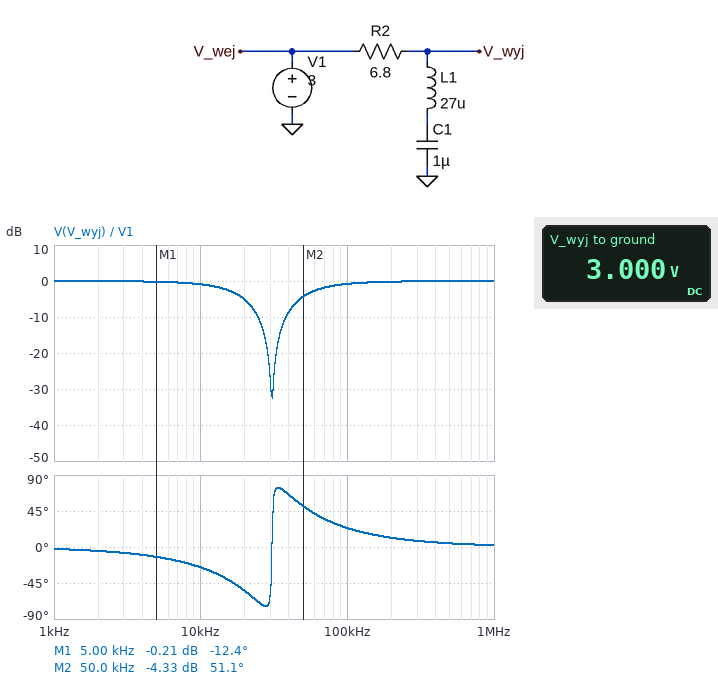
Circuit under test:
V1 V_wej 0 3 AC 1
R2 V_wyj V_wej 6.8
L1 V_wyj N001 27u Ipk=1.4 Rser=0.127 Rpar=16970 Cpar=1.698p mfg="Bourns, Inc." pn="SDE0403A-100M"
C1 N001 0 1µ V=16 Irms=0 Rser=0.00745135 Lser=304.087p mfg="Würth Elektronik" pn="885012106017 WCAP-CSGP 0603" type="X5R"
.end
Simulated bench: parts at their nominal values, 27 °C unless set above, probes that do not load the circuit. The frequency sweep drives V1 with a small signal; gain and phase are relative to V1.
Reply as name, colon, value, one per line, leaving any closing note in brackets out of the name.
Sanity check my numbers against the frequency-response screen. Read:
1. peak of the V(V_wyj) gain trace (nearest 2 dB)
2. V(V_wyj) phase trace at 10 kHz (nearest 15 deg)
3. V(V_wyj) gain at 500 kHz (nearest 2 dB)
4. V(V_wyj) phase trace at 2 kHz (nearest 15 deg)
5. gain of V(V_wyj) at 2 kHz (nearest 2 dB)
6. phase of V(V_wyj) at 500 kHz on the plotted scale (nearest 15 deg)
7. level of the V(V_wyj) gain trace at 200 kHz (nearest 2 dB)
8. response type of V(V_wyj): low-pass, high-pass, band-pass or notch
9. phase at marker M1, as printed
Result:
peak of the V(V_wyj) gain trace: 0 dB
V(V_wyj) phase trace at 10 kHz: -30 deg
V(V_wyj) gain at 500 kHz: 0 dB
V(V_wyj) phase trace at 2 kHz: 0 deg
gain of V(V_wyj) at 2 kHz: 0 dB
phase of V(V_wyj) at 500 kHz on the plotted scale: 0 deg
level of the V(V_wyj) gain trace at 200 kHz: 0 dB
response type of V(V_wyj): low-pass, high-pass, band-pass or notch: notch
phase at marker M1, as printed: -12.4 deg
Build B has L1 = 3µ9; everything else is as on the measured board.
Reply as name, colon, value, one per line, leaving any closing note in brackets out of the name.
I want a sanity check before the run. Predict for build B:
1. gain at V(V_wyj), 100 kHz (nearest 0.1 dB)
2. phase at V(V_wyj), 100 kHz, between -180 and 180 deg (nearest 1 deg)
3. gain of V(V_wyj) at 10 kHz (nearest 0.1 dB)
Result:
gain at V(V_wyj), 100 kHz: -18.1 dB
phase at V(V_wyj), 100 kHz, between -180 and 180 deg: 74 deg
gain of V(V_wyj) at 10 kHz: -0.8 dB
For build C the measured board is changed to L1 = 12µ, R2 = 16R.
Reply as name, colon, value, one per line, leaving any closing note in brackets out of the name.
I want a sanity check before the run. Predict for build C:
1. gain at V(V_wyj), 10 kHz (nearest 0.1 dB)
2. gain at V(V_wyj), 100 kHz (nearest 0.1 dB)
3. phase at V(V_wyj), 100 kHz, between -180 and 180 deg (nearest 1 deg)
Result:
gain at V(V_wyj), 10 kHz: -3.3 dB
gain at V(V_wyj), 100 kHz: -9.2 dB
phase at V(V_wyj), 100 kHz, between -180 and 180 deg: 68 deg
